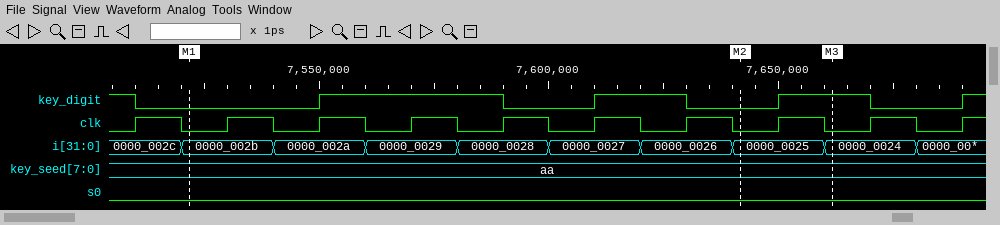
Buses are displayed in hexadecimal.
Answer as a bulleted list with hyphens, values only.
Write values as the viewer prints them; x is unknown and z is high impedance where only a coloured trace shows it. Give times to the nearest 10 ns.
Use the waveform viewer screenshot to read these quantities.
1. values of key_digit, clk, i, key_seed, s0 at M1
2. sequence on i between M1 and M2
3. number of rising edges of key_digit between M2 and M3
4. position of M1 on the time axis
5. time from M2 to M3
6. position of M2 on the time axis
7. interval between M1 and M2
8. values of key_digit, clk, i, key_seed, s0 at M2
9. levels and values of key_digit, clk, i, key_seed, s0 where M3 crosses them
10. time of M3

- key_digit=0, clk=0, i=0000_002b, key_seed=aa, s0=0
- 0000_002b, 0000_002a, 0000_0029, 0000_0028, 0000_0027, 0000_0026, 0000_0025
- 1
- 7520 ns
- 20 ns
- 7640 ns
- 120 ns
- key_digit=0, clk=0, i=0000_0025, key_seed=aa, s0=0
- key_digit=1, clk=0, i=0000_0024, key_seed=aa, s0=0
- 7660 ns
